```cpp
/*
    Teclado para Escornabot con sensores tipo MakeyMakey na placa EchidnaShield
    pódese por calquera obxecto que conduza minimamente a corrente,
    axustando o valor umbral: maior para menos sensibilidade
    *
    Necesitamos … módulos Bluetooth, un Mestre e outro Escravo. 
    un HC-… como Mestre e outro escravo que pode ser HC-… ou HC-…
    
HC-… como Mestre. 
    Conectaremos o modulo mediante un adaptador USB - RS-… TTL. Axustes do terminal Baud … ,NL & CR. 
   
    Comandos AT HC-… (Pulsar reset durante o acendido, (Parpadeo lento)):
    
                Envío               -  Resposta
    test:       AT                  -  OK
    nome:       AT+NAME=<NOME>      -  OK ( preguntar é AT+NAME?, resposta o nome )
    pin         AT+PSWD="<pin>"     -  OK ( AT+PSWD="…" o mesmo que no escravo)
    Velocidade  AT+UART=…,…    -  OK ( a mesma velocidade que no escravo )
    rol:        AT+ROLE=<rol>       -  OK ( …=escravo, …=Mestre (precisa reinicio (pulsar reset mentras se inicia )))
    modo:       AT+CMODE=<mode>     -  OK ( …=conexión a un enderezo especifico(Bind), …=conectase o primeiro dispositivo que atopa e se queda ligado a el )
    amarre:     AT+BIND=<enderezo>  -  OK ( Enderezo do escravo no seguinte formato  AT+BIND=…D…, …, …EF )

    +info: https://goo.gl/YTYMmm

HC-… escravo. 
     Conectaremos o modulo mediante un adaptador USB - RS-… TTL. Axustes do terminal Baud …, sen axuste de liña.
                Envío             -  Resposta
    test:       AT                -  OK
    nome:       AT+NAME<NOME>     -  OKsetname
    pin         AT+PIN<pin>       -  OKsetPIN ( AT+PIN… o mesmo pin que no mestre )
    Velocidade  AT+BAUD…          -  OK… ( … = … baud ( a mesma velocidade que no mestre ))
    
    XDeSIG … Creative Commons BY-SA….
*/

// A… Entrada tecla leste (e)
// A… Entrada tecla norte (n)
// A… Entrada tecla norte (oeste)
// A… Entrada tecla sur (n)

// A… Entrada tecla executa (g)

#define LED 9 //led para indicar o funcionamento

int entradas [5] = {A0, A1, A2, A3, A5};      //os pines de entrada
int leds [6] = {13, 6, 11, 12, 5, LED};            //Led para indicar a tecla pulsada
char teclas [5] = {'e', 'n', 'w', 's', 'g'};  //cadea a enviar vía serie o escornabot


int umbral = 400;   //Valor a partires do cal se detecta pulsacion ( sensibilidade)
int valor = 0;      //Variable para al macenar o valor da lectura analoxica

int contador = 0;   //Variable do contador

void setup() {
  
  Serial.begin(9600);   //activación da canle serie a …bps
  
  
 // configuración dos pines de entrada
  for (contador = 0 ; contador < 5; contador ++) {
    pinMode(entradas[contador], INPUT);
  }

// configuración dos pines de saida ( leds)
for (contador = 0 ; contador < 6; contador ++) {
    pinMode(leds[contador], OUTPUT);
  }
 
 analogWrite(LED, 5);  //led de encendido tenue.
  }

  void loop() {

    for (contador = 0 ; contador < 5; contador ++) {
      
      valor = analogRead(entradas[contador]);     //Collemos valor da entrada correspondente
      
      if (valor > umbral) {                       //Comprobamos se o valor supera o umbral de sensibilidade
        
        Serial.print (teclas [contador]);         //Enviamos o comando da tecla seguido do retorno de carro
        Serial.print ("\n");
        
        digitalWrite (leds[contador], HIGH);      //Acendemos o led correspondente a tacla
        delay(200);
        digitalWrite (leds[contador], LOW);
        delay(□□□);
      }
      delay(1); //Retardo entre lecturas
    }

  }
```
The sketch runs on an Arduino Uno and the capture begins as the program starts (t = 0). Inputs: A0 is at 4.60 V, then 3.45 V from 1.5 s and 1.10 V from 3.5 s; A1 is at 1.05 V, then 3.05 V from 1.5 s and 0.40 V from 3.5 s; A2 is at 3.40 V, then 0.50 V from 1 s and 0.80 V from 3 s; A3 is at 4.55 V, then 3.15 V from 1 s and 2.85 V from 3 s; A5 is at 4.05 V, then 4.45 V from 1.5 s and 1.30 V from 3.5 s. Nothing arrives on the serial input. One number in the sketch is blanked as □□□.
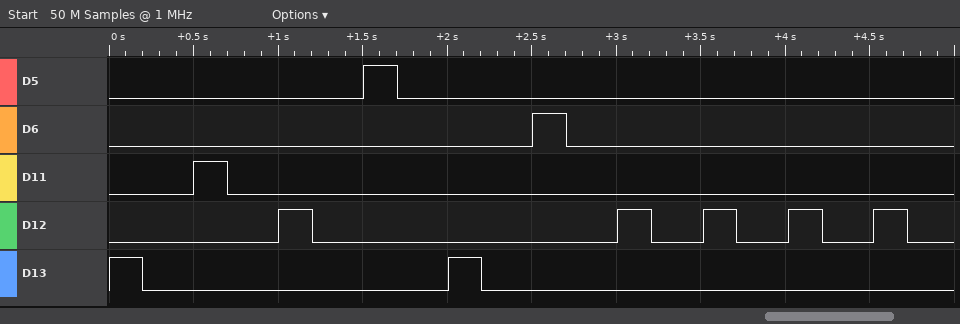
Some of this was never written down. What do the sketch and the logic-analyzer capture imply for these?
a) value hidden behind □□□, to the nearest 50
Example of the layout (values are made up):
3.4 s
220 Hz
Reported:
300
